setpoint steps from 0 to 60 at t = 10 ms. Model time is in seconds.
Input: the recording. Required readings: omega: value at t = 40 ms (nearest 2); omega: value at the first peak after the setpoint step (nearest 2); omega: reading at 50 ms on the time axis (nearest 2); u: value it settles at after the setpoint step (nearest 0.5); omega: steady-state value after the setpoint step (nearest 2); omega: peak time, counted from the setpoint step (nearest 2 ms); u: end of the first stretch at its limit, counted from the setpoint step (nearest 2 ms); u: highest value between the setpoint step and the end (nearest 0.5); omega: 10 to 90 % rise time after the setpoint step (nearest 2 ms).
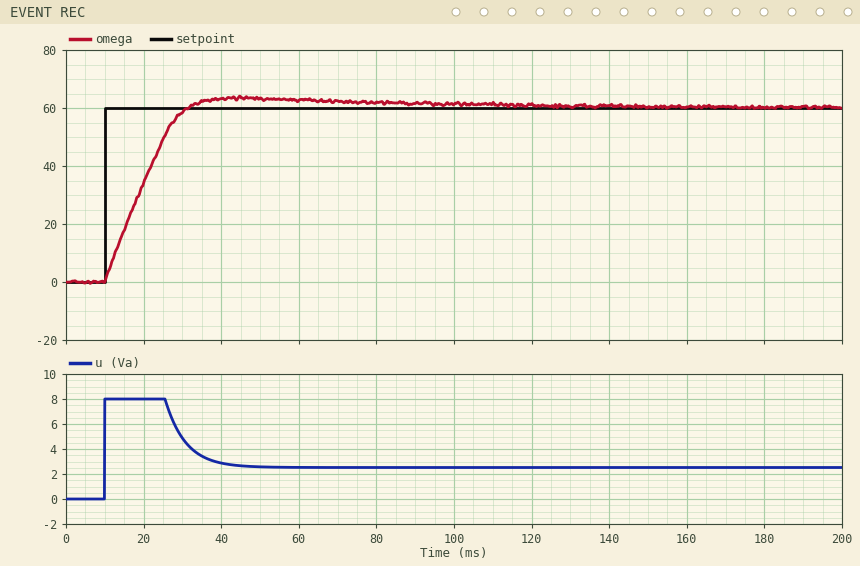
64
64
64
2.5
60
34 ms
16 ms
8.0
16 ms
